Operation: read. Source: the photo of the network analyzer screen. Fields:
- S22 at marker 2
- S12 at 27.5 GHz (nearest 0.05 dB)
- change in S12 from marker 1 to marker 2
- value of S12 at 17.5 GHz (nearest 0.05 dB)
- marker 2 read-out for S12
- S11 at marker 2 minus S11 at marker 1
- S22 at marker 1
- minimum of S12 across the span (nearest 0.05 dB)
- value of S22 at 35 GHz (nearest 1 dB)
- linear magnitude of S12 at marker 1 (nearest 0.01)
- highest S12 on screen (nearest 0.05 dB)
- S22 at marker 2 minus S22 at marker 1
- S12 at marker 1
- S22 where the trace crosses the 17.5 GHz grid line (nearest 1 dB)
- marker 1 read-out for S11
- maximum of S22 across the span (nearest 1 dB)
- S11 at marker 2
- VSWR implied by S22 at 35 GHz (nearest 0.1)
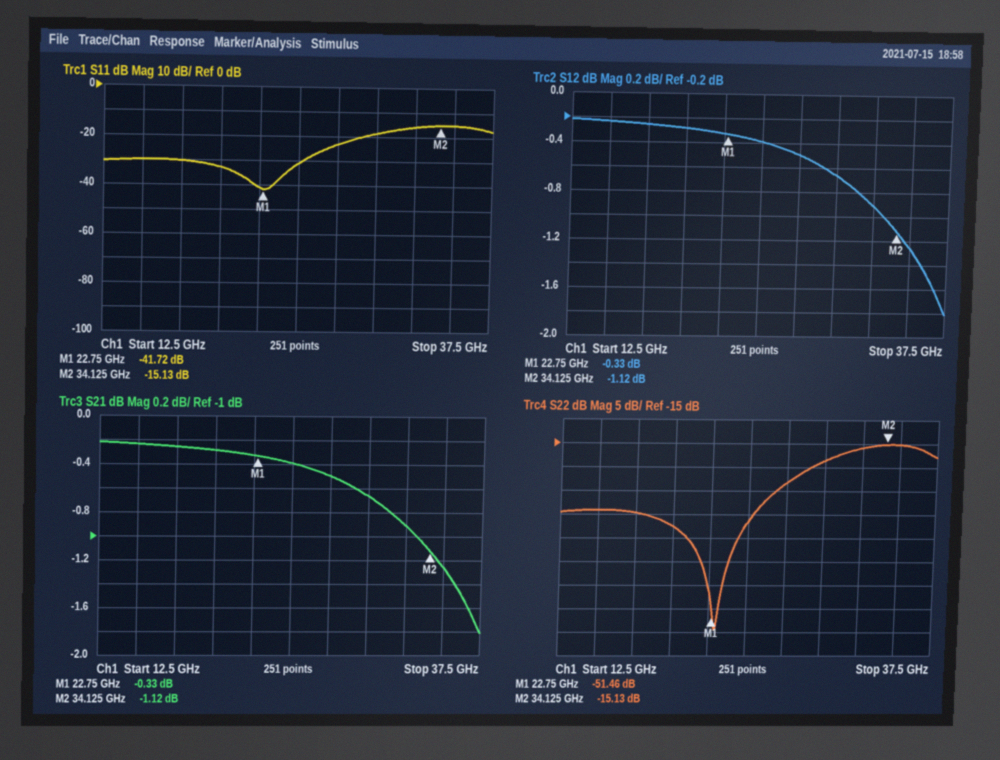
-15.13 dB
-0.50 dB
-0.79 dB
-0.25 dB
-1.12 dB
26.59 dB
-51.46 dB
-1.80 dB
-15 dB
0.96
-0.20 dB
36.33 dB
-0.33 dB
-30 dB
-41.72 dB
-15 dB
-15.13 dB
1.4
